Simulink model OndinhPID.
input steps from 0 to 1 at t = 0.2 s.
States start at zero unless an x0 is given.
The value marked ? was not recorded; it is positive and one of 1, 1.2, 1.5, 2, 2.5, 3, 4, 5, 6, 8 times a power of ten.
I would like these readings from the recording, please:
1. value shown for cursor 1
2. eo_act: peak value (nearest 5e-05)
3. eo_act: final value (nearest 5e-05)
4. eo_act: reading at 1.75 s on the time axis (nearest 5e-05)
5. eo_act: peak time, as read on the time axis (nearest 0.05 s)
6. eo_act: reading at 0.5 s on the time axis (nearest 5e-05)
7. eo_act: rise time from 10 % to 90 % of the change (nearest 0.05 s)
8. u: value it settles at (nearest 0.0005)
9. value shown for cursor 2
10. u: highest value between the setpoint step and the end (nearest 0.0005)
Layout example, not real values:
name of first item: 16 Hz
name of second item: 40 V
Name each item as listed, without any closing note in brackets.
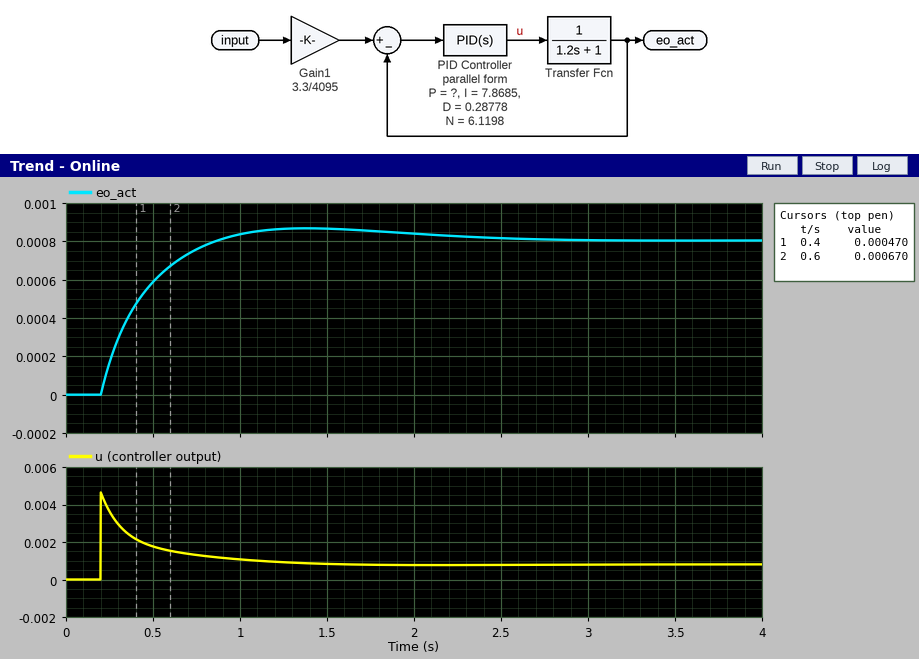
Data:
value shown for cursor 1: 0.000470
eo_act: peak value: 0.00085
eo_act: final value: 0.00080
eo_act: reading at 1.75 s on the time axis: 0.00085
eo_act: peak time, as read on the time axis: 1.40 s
eo_act: reading at 0.5 s on the time axis: 0.00060
eo_act: rise time from 10 % to 90 % of the change: 0.45 s
u: value it settles at: 0.0010
value shown for cursor 2: 0.000670
u: highest value between the setpoint step and the end: 0.0045
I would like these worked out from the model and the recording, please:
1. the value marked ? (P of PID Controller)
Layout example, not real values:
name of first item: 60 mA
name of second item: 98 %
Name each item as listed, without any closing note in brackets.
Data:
the value marked ?: 4
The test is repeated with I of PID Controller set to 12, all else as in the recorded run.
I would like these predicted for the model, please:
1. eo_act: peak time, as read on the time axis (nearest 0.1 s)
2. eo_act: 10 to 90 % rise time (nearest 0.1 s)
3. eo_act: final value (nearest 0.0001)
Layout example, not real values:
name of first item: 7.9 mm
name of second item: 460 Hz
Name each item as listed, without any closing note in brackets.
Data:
eo_act: peak time, as read on the time axis: 1.1 s
eo_act: 10 to 90 % rise time: 0.4 s
eo_act: final value: 0.0008
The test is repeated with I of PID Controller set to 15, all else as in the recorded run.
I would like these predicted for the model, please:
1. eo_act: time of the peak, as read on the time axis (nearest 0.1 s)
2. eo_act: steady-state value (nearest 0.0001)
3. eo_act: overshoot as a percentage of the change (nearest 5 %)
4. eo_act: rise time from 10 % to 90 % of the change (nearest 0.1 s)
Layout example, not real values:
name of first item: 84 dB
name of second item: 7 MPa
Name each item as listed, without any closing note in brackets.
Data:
eo_act: time of the peak, as read on the time axis: 1.0 s
eo_act: steady-state value: 0.0008
eo_act: overshoot as a percentage of the change: 15 %
eo_act: rise time from 10 % to 90 % of the change: 0.3 s
